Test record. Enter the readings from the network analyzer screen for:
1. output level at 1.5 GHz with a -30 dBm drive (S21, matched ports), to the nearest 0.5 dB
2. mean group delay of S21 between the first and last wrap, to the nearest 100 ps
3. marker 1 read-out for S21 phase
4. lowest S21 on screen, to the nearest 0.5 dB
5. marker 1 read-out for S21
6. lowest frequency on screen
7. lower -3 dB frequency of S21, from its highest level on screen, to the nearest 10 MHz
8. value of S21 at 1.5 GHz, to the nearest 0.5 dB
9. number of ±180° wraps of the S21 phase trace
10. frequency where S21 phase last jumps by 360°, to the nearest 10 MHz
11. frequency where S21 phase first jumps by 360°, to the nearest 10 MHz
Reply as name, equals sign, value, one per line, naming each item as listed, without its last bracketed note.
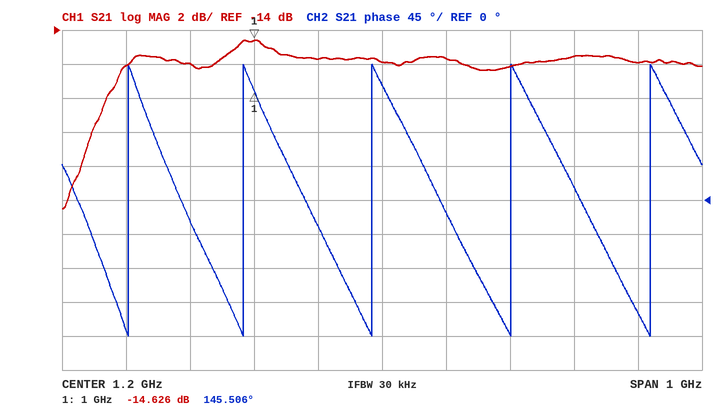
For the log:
output level at 1.5 GHz with a -30 dBm drive (S21, matched ports), to the nearest 0.5 dB = -45.5 dBm
mean group delay of S21 between the first and last wrap, to the nearest 100 ps = 4.9 ns
marker 1 read-out for S21 phase = 145.506°
lowest S21 on screen, to the nearest 0.5 dB = -24.5 dB
marker 1 read-out for S21 = -14.626 dB
lowest frequency on screen = 700 MHz
lower -3 dB frequency of S21, from its highest level on screen, to the nearest 10 MHz = 780 MHz
value of S21 at 1.5 GHz, to the nearest 0.5 dB = -15.5 dB
number of ±180° wraps of the S21 phase trace = 5
frequency where S21 phase last jumps by 360°, to the nearest 10 MHz = 1.62 GHz
frequency where S21 phase first jumps by 360°, to the nearest 10 MHz = 800 MHz
